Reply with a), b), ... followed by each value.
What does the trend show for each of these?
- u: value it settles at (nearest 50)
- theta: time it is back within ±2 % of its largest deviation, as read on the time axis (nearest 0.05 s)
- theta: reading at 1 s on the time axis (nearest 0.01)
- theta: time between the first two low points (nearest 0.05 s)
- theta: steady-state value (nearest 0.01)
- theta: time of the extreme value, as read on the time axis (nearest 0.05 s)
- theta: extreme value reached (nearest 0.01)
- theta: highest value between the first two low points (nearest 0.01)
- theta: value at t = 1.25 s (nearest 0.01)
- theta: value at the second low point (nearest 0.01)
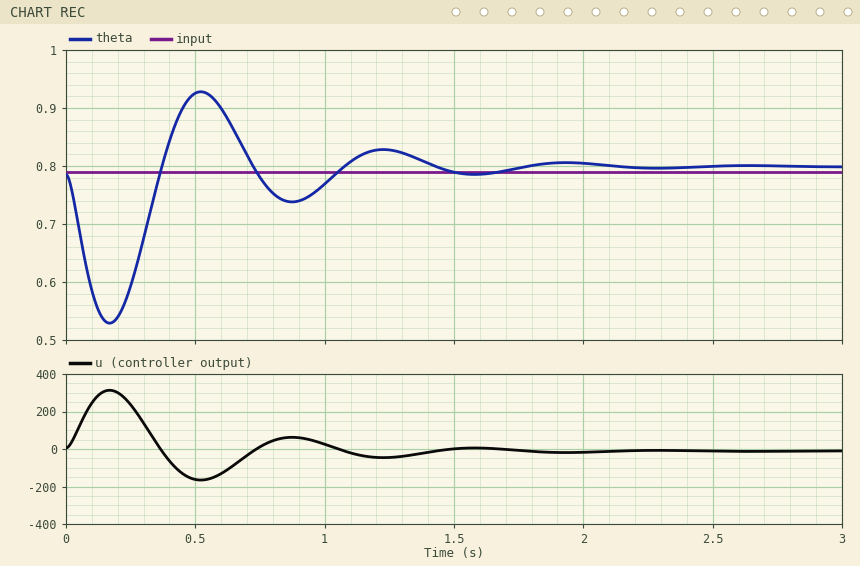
a) 0
b) 2.00 s
c) 0.77
d) 0.70 s
e) 0.80
f) 0.15 s
g) 0.53
h) 0.93
i) 0.83
j) 0.74
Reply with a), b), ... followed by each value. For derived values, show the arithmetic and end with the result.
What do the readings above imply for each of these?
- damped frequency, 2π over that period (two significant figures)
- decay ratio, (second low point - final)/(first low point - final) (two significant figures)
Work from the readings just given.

a) 2π / 0.7 = 9.0 rad/s
b) (0.74 - 0.8) / (0.53 - 0.8) = 0.22
